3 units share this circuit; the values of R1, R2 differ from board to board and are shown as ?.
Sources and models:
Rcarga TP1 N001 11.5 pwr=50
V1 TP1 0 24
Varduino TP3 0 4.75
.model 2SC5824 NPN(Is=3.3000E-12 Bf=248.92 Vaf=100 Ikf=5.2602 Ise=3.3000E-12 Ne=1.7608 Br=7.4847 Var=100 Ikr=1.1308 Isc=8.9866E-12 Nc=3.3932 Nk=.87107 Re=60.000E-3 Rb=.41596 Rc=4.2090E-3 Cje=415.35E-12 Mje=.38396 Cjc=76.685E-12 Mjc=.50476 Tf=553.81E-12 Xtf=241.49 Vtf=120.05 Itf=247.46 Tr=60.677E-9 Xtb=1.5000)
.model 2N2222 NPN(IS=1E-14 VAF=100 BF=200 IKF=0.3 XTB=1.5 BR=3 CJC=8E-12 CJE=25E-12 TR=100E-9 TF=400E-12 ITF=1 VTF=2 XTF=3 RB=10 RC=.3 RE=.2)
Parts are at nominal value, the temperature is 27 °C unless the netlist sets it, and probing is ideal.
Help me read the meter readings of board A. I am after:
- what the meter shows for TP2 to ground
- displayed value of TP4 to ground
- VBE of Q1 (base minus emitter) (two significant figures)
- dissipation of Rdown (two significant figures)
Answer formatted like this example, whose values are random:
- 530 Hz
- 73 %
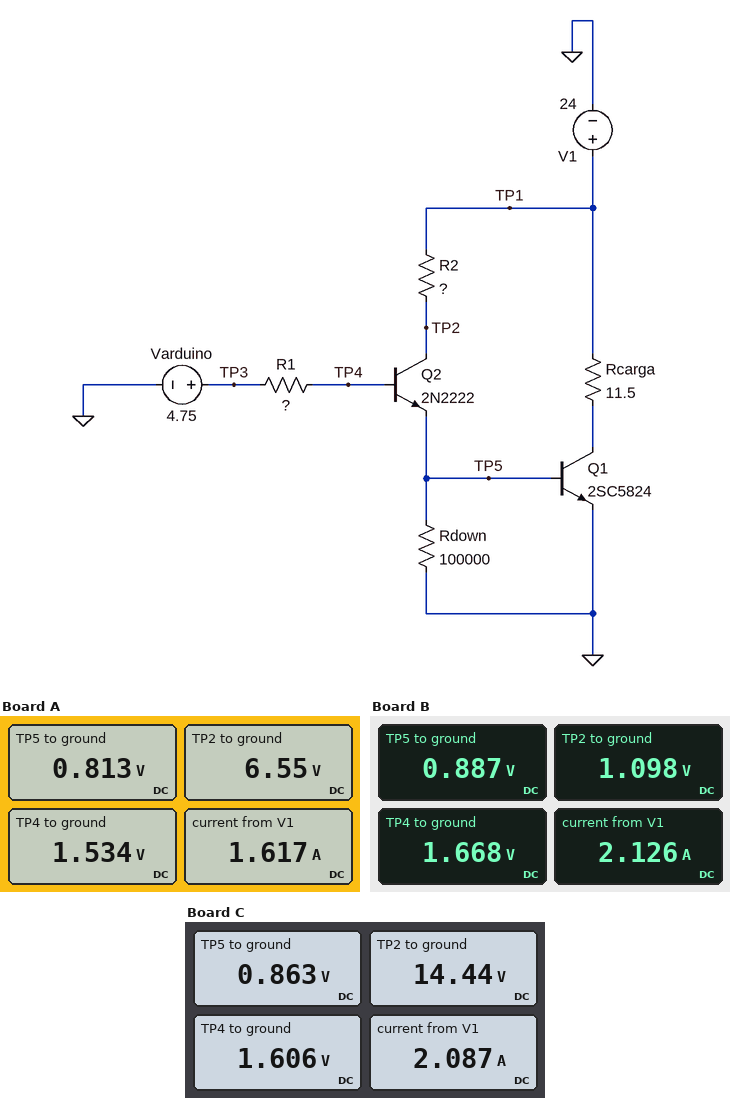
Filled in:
- 6.55 V
- 1.534 V
- 810 mV
- 6.6 µW
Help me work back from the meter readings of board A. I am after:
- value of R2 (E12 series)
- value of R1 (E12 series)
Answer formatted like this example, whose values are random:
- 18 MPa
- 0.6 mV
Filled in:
- 1.5 kΩ
- 56 kΩ
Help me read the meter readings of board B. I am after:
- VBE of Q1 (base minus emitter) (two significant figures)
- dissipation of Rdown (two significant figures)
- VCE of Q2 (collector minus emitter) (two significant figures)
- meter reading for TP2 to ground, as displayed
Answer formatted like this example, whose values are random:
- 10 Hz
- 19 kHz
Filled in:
- 890 mV
- 7.9 µW
- 210 mV
- 1.098 V
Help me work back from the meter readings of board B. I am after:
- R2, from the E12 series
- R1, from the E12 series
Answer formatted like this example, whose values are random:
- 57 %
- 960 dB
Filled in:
- 390 Ω
- 8.2 kΩ
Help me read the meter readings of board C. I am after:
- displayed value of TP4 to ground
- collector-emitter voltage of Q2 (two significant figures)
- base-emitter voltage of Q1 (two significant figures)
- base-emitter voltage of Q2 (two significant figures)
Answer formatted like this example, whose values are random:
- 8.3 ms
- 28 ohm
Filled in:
- 1.606 V
- 14 V
- 860 mV
- 740 mV
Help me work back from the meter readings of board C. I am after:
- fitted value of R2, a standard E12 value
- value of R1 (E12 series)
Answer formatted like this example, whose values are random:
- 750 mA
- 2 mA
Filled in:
- 390 Ω
- 27 kΩ
